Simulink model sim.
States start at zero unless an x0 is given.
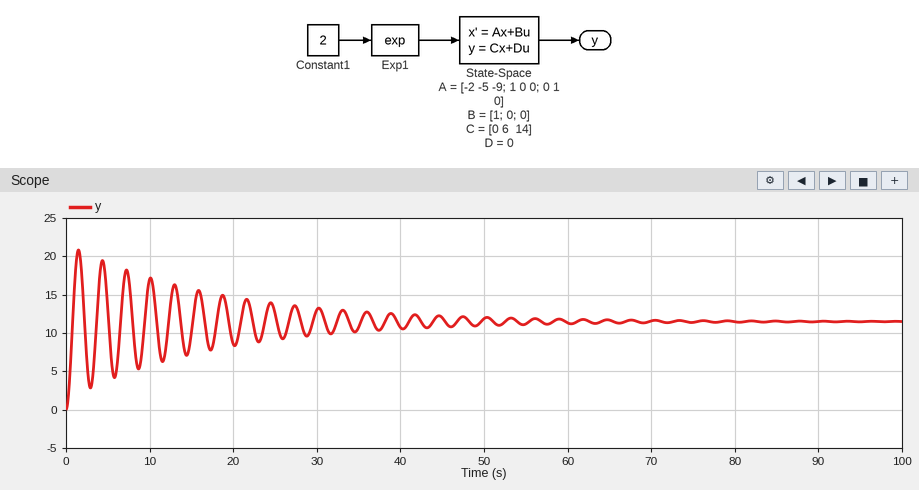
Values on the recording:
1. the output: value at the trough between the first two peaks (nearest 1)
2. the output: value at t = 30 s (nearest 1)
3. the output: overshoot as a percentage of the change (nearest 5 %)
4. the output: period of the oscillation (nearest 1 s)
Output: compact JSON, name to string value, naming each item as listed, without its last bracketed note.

{"the output: value at the trough between the first two peaks": "3", "the output: value at t = 30 s": "13", "the output: overshoot as a percentage of the change": "80 %", "the output: period of the oscillation": "3 s"}
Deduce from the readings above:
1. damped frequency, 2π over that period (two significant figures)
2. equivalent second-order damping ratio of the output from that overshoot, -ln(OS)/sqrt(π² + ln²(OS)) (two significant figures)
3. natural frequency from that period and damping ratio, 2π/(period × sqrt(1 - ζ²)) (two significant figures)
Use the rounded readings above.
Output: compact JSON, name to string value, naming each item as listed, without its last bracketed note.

{"damped frequency, 2π over that period": "2.1 rad/s", "equivalent second-order damping ratio of the output from that overshoot, -ln(OS)/sqrt(π² + ln²(OS))": "0.071", "natural frequency from that period and damping ratio, 2π/(period × sqrt(1 - ζ²))": "2.1 rad/s"}
